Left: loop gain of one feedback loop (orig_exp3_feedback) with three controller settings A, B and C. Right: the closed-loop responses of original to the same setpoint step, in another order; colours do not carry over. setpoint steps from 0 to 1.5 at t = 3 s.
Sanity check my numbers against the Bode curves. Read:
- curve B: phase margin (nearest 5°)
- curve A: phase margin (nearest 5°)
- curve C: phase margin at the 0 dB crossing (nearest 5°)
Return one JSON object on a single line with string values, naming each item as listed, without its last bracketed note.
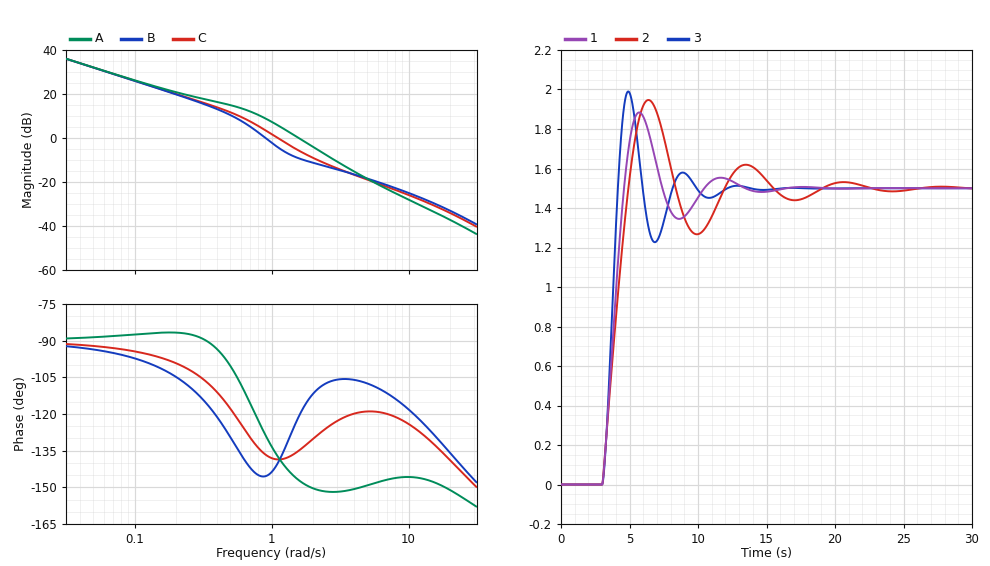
{"curve B: phase margin": "35°", "curve A: phase margin": "35°", "curve C: phase margin at the 0 dB crossing": "40°"}
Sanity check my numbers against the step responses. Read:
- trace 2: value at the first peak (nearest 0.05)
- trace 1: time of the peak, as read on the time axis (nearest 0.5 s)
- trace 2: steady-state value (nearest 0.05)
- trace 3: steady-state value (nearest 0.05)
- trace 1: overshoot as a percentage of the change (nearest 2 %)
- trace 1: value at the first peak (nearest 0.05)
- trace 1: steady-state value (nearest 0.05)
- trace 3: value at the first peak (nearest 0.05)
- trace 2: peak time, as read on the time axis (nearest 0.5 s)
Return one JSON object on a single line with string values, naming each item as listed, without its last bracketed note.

{"trace 2: value at the first peak": "1.95", "trace 1: time of the peak, as read on the time axis": "5.5 s", "trace 2: steady-state value": "1.50", "trace 3: steady-state value": "1.50", "trace 1: overshoot as a percentage of the change": "26 %", "trace 1: value at the first peak": "1.90", "trace 1: steady-state value": "1.50", "trace 3: value at the first peak": "2.00", "trace 2: peak time, as read on the time axis": "6.5 s"}
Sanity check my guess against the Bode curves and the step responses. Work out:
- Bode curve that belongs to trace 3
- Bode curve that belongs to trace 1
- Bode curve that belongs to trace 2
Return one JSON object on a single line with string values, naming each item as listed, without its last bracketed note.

{"Bode curve that belongs to trace 3": "A", "Bode curve that belongs to trace 1": "C", "Bode curve that belongs to trace 2": "B"}
